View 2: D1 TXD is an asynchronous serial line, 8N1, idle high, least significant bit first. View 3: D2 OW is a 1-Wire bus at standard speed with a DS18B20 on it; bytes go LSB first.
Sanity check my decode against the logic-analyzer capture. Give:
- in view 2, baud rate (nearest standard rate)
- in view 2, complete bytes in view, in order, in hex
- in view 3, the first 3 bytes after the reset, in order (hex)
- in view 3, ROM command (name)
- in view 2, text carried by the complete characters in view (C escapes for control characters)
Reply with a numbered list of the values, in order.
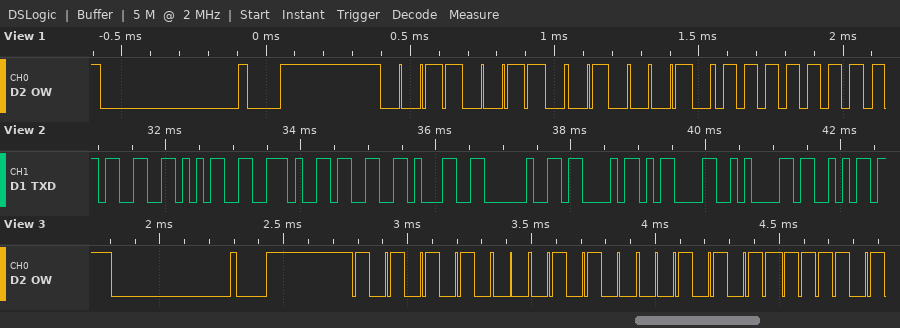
1. 9600 baud
2. 33 35 2E 33 31 20 43 0D 0A 53
3. 55 28 D4
4. Match ROM
5. "35.31 C\r\nS"
